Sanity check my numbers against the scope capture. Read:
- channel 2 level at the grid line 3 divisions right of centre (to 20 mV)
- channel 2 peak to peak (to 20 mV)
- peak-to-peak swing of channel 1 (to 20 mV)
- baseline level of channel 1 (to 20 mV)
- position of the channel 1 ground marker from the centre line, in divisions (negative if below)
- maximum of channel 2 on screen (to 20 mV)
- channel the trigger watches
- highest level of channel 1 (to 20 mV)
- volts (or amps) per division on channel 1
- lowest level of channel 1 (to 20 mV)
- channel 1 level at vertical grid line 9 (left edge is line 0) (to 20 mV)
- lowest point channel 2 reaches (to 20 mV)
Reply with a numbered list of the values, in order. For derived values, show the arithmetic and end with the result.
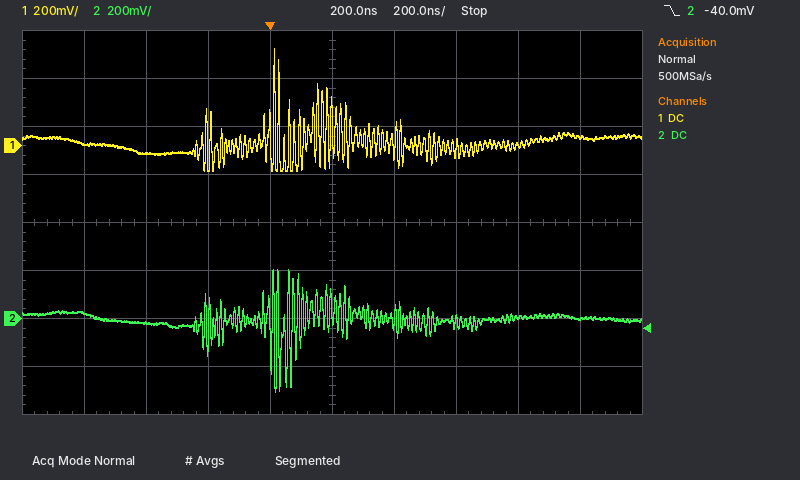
1. 0 mV
2. 200 mV − (-300 mV) = 500 mV
3. 400 mV − (-100 mV) = 500 mV
4. 20 mV
5. +1.6 div
6. 200 mV
7. channel 2
8. 400 mV
9. 200 mV
10. -100 mV
11. 40 mV
12. -300 mV
